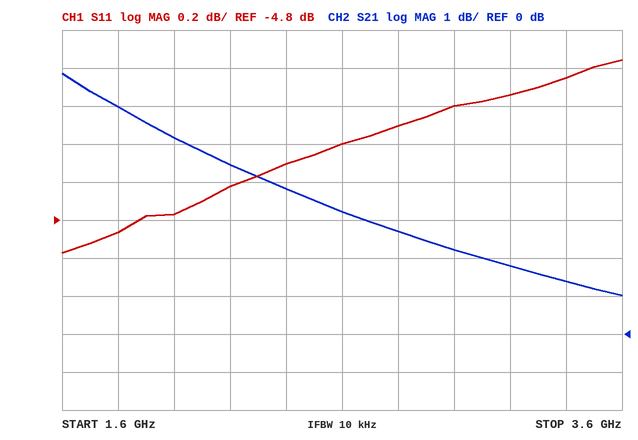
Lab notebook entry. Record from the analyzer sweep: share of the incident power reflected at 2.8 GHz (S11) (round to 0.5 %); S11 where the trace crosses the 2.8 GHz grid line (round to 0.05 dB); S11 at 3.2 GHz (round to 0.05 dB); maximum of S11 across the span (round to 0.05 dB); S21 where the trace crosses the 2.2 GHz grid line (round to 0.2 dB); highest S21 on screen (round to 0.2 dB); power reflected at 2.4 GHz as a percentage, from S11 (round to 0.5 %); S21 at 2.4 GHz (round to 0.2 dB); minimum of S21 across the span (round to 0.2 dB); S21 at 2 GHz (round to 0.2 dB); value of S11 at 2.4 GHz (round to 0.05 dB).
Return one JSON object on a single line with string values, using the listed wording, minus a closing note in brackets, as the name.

{"share of the incident power reflected at 2.8 GHz (S11)": "37.0 %", "S11 where the trace crosses the 2.8 GHz grid line": "-4.30 dB", "S11 at 3.2 GHz": "-4.15 dB", "maximum of S11 across the span": "-3.95 dB", "S21 where the trace crosses the 2.2 GHz grid line": "4.4 dB", "highest S21 on screen": "6.8 dB", "power reflected at 2.4 GHz as a percentage, from S11": "35.5 %", "S21 at 2.4 GHz": "3.8 dB", "minimum of S21 across the span": "1.0 dB", "S21 at 2 GHz": "5.2 dB", "value of S11 at 2.4 GHz": "-4.50 dB"}
